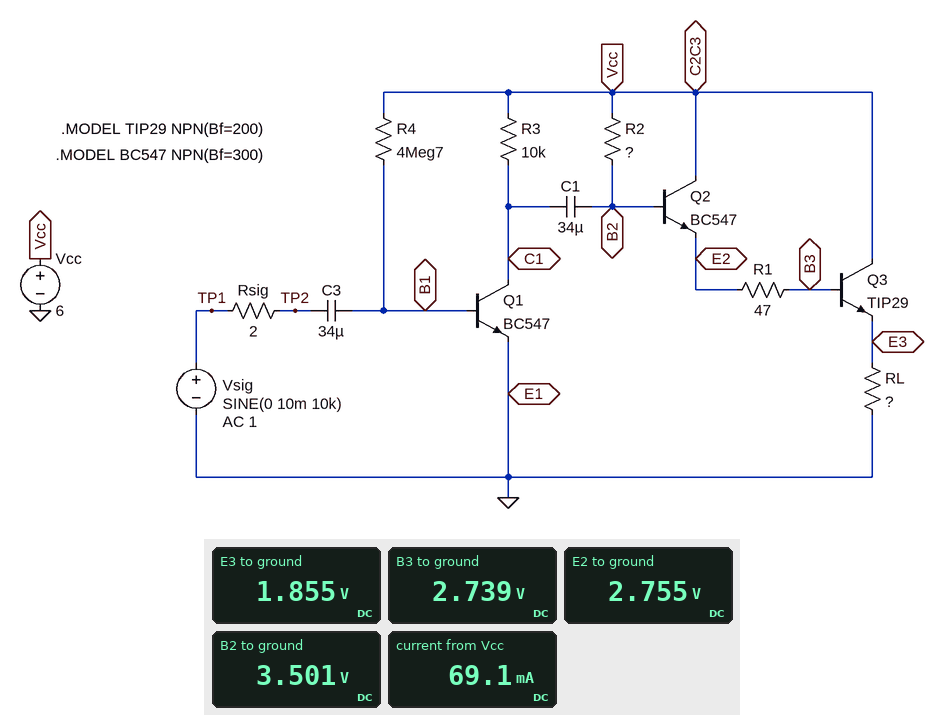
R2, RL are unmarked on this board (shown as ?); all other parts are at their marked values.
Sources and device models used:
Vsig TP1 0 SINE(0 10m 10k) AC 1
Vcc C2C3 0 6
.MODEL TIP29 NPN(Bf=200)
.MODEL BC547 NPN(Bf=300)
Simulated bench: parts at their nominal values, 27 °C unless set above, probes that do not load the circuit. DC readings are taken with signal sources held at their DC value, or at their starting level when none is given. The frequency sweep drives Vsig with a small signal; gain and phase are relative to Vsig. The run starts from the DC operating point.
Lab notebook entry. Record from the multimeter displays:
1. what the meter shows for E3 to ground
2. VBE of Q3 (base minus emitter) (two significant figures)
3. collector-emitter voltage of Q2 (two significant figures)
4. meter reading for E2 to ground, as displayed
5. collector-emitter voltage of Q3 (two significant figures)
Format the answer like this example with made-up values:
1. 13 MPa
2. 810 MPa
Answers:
1. 1.855 V
2. 880 mV
3. 3.2 V
4. 2.755 V
5. 4.1 V
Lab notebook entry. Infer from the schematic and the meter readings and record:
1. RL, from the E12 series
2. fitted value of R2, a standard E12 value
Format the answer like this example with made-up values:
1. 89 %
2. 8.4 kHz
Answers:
1. 27 Ω
2. 2.2 MΩ
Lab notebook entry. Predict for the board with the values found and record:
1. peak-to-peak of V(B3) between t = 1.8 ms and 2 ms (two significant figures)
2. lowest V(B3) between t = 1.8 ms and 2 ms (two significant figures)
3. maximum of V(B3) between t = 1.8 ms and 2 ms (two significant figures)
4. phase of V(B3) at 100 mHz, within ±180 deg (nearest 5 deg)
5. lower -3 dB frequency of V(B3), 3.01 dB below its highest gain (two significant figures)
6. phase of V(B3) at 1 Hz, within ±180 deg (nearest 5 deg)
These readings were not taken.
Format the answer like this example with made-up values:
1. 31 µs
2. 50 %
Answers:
1. 2.6 V
2. 1.2 V
3. 3.8 V
4. -115 deg
5. 200 mHz
6. -170 deg
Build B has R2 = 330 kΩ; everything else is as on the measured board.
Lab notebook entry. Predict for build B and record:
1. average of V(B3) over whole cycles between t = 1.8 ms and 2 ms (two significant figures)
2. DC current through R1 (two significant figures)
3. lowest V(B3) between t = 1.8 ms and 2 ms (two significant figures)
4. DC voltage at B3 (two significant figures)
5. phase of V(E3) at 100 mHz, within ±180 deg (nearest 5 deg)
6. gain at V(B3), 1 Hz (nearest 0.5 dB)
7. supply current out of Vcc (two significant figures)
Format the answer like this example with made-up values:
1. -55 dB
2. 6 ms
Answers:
1. 4.4 V
2. 660 µA
3. 3.0 V
4. 4.5 V
5. -105 deg
6. 41.5 dB
7. 130 mA
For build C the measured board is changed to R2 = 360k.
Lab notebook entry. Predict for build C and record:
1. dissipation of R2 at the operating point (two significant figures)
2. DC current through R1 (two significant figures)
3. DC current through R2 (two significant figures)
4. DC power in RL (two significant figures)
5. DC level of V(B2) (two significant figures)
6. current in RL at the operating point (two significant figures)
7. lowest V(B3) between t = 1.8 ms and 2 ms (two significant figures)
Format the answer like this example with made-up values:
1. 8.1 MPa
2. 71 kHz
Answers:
1. 1.7 µW
2. 650 µA
3. 2.2 µA
4. 460 mW
5. 5.2 V
6. 130 mA
7. 2.9 V
